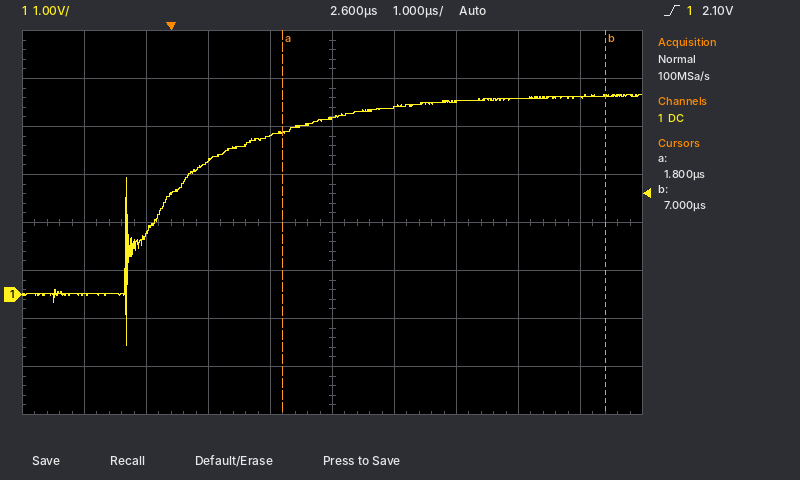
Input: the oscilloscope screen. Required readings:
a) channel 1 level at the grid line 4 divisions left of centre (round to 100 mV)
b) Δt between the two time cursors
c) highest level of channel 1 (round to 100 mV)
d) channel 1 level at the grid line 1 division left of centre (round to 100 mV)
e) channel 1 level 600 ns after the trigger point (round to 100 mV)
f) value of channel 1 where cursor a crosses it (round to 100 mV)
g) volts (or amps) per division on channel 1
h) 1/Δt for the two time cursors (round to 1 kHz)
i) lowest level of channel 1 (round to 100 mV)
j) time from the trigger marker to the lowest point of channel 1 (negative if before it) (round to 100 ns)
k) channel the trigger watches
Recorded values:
0.0 V
5.2 µs
4.2 V
3.3 V
2.8 V
3.4 V
1 V
192 kHz
-1.1 V
-700 ns
channel 1
